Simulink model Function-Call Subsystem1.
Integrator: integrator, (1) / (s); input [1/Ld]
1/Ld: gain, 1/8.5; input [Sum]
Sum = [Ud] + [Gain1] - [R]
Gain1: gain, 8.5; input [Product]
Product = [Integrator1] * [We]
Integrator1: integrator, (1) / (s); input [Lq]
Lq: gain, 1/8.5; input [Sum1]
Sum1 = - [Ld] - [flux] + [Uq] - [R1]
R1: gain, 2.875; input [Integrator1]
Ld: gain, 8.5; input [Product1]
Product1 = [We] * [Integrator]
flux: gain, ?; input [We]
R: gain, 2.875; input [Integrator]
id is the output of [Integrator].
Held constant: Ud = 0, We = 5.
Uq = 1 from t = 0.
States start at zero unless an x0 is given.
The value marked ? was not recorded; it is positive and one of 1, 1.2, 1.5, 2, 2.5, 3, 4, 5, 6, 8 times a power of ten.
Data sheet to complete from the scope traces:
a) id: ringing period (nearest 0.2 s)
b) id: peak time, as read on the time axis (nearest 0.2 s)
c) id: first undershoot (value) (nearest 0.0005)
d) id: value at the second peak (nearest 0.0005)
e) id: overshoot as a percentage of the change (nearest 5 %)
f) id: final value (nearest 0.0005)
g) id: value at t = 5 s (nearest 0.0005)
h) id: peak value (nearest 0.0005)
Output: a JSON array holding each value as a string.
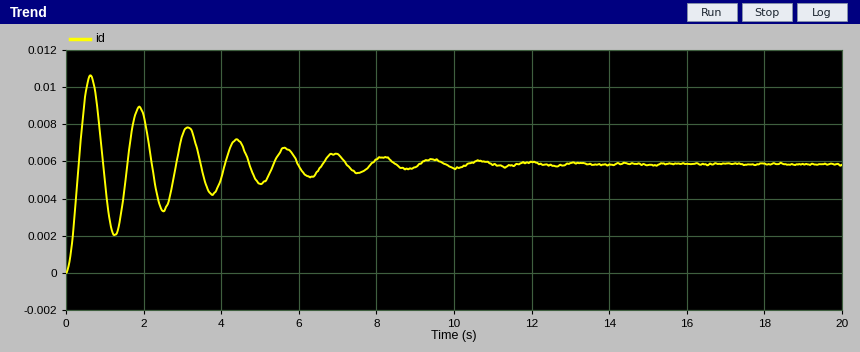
["1.2 s", "0.6 s", "0.0020", "0.0090", "80 %", "0.0060", "0.0050", "0.0105"]
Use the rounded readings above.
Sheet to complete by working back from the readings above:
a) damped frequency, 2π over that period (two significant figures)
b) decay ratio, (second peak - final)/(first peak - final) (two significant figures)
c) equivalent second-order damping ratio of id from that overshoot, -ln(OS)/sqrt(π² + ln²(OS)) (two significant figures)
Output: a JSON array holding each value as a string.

["5.2 rad/s", "0.67", "0.071"]
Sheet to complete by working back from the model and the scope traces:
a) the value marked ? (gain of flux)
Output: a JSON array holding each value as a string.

["0.15"]
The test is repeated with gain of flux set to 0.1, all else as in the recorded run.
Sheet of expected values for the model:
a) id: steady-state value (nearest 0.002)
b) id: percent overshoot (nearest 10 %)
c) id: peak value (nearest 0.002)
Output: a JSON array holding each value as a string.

["0.012", "80 %", "0.022"]
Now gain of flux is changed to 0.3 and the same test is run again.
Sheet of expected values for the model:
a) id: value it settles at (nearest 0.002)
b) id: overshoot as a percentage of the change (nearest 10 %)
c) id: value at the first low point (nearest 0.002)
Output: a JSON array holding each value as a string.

["-0.012", "80 %", "-0.022"]
